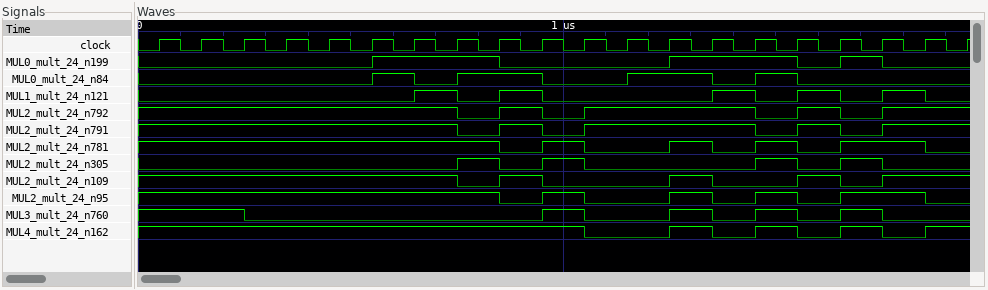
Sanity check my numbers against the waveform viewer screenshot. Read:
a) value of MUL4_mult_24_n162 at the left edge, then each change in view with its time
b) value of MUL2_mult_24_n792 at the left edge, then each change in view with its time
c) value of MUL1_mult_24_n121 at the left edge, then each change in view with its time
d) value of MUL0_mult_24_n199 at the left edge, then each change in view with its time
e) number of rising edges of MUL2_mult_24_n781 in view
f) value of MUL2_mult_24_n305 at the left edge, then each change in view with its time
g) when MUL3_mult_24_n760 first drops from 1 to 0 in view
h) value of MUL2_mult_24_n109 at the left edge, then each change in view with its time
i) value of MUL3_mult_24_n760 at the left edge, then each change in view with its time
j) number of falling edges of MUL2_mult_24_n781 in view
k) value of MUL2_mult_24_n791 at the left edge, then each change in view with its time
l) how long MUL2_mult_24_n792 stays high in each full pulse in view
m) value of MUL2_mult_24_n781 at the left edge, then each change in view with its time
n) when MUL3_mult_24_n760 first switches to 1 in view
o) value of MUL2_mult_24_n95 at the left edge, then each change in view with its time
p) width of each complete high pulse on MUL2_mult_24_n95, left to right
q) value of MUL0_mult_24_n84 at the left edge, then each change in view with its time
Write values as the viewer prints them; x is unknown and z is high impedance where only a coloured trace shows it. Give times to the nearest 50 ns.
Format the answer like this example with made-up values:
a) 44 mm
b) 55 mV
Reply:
a) 1, 0 at 1050 ns, 1 at 1250 ns, 0 at 1350 ns, 1 at 1450 ns, 0 at 1550 ns, 1 at 1650 ns, 0 at 1750 ns, 1 at 1850 ns
b) 1, 0 at 750 ns, 1 at 850 ns, 0 at 950 ns, 1 at 1050 ns, 0 at 1450 ns, 1 at 1550 ns, 0 at 1650 ns, 1 at 1750 ns
c) 0, 1 at 650 ns, 0 at 750 ns, 1 at 850 ns, 0 at 950 ns, 1 at 1350 ns, 0 at 1450 ns, 1 at 1550 ns, 0 at 1650 ns, 1 at 1750 ns, 0 at 1850 ns
d) 0, 1 at 550 ns, 0 at 850 ns, 1 at 1250 ns, 0 at 1550 ns, 1 at 1650 ns, 0 at 1750 ns
e) 4
f) 0, 1 at 750 ns, 0 at 850 ns, 1 at 950 ns, 0 at 1050 ns, 1 at 1450 ns, 0 at 1550 ns, 1 at 1650 ns, 0 at 1750 ns
g) 250 ns
h) 1, 0 at 750 ns, 1 at 850 ns, 0 at 950 ns, 1 at 1250 ns, 0 at 1350 ns, 1 at 1550 ns, 0 at 1650 ns, 1 at 1750 ns
i) 1, 0 at 250 ns, 1 at 950 ns, 0 at 1050 ns, 1 at 1250 ns, 0 at 1350 ns, 1 at 1450 ns, 0 at 1550 ns, 1 at 1650 ns, 0 at 1750 ns
j) 5
k) 1, 0 at 750 ns, 1 at 850 ns, 0 at 950 ns, 1 at 1050 ns, 0 at 1450 ns, 1 at 1550 ns, 0 at 1650 ns, 1 at 1750 ns
l) 100 ns, 400 ns, 100 ns
m) 1, 0 at 850 ns, 1 at 950 ns, 0 at 1050 ns, 1 at 1250 ns, 0 at 1350 ns, 1 at 1450 ns, 0 at 1550 ns, 1 at 1650 ns, 0 at 1850 ns
n) 950 ns
o) 1, 0 at 850 ns, 1 at 950 ns, 0 at 1050 ns, 1 at 1250 ns, 0 at 1350 ns, 1 at 1450 ns, 0 at 1550 ns, 1 at 1650 ns, 0 at 1850 ns
p) 100 ns, 100 ns, 100 ns, 200 ns
q) 0, 1 at 550 ns, 0 at 650 ns, 1 at 750 ns, 0 at 950 ns, 1 at 1150 ns, 0 at 1350 ns, 1 at 1450 ns, 0 at 1550 ns
